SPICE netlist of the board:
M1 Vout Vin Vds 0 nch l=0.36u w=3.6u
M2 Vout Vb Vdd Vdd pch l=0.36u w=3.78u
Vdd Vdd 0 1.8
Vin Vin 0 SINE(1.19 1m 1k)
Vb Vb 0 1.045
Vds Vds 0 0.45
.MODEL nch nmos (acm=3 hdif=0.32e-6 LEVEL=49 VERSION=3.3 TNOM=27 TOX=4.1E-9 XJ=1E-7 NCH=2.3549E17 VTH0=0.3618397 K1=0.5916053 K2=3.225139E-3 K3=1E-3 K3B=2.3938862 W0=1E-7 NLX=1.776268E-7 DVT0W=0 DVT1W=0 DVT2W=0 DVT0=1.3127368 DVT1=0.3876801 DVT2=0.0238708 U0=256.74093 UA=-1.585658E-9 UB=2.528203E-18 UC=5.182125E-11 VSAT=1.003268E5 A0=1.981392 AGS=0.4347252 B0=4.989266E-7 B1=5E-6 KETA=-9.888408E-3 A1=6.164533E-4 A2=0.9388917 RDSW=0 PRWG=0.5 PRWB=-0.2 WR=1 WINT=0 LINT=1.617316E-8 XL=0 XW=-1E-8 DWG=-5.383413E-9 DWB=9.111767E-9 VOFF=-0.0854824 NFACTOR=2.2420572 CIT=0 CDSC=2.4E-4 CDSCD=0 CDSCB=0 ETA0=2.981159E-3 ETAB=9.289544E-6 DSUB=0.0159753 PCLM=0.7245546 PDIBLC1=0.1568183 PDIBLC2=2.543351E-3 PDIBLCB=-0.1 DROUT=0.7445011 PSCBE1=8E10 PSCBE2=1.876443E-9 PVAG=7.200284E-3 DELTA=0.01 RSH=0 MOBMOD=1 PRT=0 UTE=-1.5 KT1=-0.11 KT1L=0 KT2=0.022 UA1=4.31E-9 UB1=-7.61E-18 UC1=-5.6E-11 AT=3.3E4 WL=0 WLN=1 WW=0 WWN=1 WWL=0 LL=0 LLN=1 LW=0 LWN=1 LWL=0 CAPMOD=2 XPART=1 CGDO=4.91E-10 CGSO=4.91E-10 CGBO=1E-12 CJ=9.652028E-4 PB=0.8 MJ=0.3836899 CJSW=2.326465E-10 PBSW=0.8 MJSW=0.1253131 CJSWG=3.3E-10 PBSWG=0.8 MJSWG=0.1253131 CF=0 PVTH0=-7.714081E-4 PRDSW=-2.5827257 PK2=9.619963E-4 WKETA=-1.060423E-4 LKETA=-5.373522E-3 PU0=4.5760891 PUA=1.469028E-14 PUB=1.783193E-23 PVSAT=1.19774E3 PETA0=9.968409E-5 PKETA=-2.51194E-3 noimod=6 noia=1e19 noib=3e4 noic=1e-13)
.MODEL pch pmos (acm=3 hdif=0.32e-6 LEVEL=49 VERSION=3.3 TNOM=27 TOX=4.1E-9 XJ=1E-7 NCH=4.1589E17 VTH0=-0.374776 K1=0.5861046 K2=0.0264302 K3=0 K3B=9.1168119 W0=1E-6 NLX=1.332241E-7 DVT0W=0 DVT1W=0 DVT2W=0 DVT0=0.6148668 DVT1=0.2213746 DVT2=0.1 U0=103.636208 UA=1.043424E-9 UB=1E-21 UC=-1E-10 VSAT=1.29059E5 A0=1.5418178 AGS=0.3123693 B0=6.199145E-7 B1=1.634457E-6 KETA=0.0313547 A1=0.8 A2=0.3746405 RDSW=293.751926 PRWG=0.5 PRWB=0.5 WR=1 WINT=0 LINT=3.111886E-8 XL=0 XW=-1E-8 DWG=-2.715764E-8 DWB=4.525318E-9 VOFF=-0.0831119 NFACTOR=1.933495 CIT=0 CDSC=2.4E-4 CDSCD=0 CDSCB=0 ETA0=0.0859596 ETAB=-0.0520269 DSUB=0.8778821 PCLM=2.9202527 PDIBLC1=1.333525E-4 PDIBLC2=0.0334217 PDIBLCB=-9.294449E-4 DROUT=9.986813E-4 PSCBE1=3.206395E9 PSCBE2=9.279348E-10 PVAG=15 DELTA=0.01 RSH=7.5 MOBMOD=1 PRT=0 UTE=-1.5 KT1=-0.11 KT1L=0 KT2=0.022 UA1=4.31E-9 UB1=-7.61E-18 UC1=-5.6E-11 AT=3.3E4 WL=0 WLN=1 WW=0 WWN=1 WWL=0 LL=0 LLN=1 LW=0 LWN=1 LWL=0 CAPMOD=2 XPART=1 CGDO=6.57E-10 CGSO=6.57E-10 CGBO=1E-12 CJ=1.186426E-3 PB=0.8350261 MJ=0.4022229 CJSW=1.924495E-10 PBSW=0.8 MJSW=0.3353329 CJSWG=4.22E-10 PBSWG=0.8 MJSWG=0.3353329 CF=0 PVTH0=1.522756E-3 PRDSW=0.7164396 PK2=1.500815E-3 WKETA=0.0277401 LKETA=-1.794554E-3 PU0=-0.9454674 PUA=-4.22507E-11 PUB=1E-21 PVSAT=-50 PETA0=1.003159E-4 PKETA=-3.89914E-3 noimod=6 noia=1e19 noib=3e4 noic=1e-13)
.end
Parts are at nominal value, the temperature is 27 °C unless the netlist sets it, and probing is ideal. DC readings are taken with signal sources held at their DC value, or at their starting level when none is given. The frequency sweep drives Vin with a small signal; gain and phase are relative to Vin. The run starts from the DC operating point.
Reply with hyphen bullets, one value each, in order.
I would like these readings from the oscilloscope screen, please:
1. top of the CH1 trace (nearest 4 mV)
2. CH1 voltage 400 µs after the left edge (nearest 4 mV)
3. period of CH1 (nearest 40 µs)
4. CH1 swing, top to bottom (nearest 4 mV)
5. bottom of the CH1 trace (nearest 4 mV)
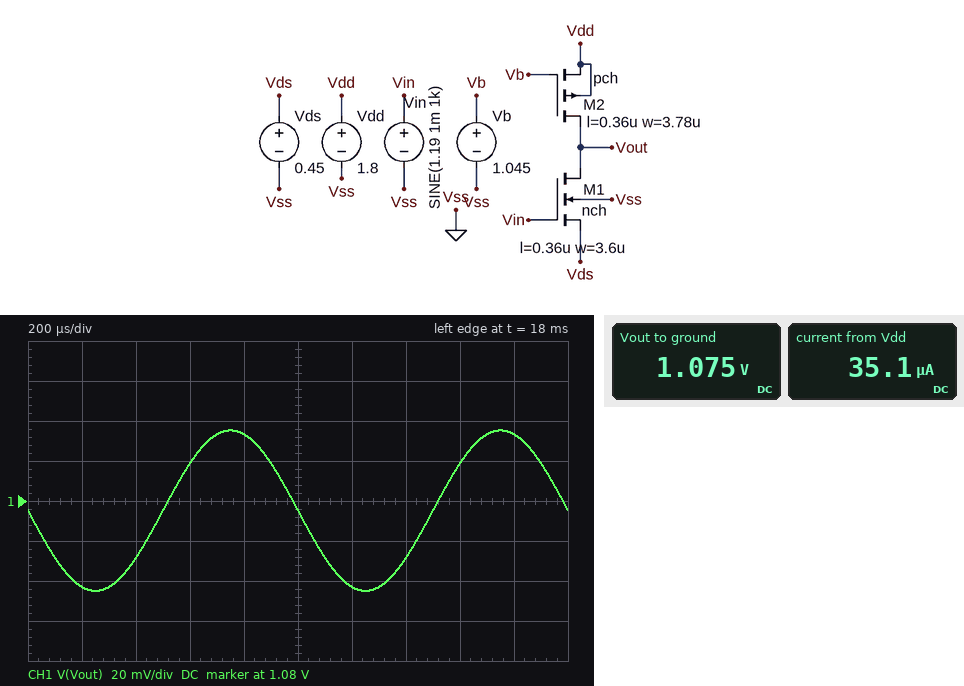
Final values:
- 1.116 V
- 1.052 V
- 1.00 ms
- 80 mV
- 1.036 V
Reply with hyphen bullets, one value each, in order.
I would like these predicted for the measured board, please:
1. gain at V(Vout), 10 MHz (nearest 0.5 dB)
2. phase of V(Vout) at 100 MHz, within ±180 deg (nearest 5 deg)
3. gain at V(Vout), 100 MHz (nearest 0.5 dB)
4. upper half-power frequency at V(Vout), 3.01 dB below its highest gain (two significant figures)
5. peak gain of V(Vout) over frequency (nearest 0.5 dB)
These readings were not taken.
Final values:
- 32.0 dB
- 145 deg
- 30.0 dB
- 140 MHz
- 32.0 dB
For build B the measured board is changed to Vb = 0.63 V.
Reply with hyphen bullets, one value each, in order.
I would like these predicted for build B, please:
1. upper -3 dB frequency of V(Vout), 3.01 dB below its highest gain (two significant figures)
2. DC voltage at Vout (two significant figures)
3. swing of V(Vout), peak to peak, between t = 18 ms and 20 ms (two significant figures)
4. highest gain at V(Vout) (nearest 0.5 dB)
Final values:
- 2.9 GHz
- 1.7 V
- 1.9 mV
- -0.5 dB
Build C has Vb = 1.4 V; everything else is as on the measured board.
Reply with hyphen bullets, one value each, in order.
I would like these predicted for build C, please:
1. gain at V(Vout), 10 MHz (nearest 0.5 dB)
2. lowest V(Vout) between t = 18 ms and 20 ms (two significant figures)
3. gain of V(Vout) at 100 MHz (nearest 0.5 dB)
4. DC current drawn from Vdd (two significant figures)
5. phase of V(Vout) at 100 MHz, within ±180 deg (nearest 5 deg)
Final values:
- -46.0 dB
- 450 mV
- -39.0 dB
- 260 nA
- 115 deg
